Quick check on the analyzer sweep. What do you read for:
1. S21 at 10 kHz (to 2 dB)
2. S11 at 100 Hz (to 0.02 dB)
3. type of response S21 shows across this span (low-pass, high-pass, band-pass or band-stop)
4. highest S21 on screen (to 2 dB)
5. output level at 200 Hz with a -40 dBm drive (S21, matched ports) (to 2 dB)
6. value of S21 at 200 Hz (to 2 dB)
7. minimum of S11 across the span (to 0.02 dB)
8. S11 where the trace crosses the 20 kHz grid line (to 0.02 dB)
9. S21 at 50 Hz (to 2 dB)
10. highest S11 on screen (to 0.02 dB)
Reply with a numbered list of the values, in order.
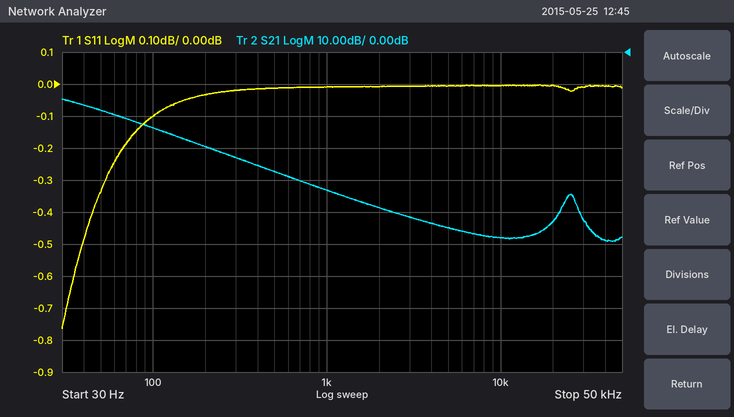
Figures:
1. -58 dB
2. -0.10 dB
3. low-pass
4. -14 dB
5. -70 dBm
6. -30 dB
7. -0.76 dB
8. 0.00 dB
9. -18 dB
10. 0.00 dB
